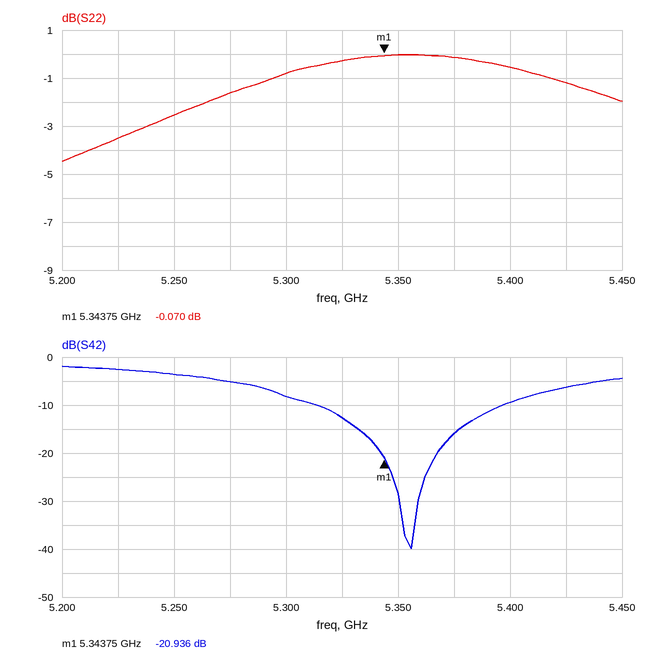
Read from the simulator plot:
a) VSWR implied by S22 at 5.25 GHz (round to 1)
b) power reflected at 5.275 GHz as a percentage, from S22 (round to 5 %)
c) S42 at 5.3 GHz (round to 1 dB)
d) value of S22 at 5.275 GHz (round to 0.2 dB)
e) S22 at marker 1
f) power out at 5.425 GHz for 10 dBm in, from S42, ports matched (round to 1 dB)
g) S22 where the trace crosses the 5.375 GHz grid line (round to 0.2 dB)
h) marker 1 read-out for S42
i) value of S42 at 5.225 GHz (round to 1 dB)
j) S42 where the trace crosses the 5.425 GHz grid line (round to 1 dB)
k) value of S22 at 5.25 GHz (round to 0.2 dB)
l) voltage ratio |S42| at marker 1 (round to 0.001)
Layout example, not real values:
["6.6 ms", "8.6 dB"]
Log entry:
["7", "70 %", "-8 dB", "-1.6 dB", "-0.070 dB", "4 dBm", "-0.2 dB", "-20.936 dB", "-3 dB", "-6 dB", "-2.6 dB", "0.090"]
